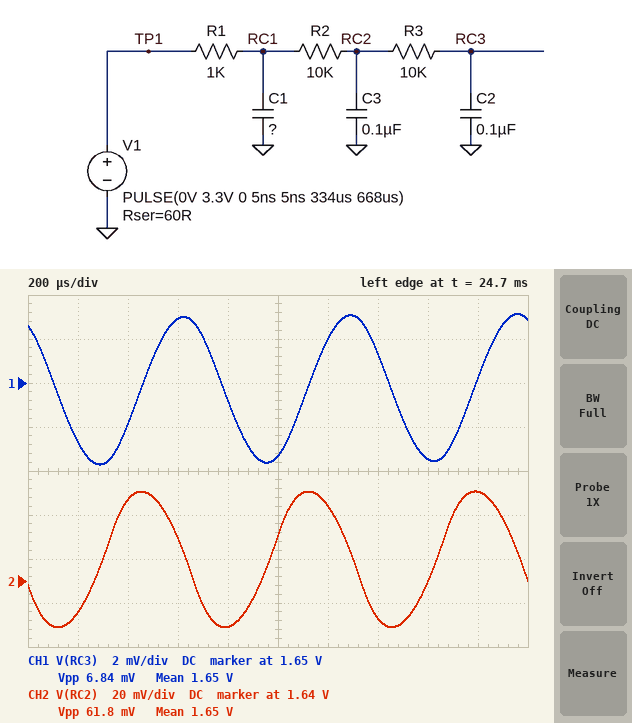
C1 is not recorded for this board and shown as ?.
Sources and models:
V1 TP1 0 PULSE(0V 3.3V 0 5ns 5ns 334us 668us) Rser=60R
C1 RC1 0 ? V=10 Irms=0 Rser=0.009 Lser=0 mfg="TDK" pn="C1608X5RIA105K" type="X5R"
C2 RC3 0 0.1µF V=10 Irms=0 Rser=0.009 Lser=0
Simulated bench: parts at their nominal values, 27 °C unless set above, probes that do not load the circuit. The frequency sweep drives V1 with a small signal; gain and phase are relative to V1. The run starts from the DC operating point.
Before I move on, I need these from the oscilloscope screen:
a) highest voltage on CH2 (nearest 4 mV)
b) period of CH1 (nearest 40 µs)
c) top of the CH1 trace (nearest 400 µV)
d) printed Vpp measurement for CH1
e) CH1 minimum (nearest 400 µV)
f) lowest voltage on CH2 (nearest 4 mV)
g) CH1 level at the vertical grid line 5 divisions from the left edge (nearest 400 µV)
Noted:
1.680 V
680 µs
1.6532 V
6.84 mV
1.6464 V
1.620 V
1.6468 V
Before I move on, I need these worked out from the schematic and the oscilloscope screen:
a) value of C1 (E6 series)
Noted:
680 nF
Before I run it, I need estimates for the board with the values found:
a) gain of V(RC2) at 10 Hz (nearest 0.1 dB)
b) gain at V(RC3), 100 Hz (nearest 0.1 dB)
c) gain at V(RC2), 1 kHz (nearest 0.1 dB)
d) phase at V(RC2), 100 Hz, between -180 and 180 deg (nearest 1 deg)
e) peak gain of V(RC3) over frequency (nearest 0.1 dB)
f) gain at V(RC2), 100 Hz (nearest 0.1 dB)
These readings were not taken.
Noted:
-0.1 dB
-7.3 dB
-30.0 dB
-65 deg
0 dB
-5.8 dB
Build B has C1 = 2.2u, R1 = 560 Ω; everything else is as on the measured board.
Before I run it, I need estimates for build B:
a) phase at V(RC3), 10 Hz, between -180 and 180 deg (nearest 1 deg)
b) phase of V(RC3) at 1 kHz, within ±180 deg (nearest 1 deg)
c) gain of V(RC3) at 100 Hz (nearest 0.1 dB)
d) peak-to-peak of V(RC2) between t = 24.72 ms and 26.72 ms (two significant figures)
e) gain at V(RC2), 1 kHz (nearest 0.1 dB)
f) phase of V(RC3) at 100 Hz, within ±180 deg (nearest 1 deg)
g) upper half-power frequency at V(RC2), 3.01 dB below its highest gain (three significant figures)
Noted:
-16 deg
123 deg
-8.6 dB
33 mV
-35.3 dB
-113 deg
52.0 Hz
